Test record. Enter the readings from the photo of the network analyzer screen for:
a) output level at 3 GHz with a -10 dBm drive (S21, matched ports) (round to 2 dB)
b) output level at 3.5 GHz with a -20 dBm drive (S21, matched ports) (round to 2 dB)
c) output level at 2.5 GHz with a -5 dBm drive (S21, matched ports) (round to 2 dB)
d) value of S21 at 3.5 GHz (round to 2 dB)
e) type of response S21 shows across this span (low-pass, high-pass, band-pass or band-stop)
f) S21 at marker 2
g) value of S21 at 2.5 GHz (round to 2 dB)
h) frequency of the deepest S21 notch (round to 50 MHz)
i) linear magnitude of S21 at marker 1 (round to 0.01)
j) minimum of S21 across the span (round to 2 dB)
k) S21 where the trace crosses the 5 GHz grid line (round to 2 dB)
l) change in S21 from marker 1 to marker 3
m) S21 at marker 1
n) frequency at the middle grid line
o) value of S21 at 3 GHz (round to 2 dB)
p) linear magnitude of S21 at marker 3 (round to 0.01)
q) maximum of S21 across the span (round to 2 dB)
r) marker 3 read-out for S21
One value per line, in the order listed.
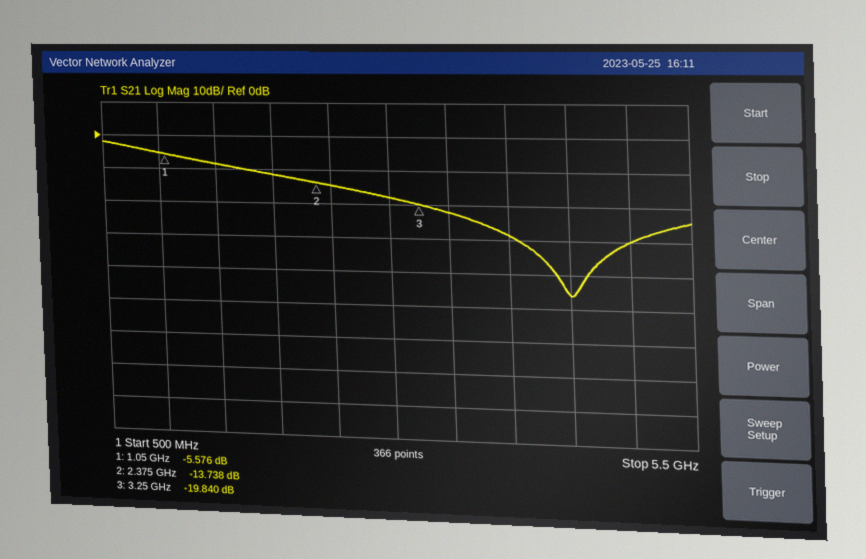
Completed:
-28 dBm
-42 dBm
-20 dBm
-22 dB
low-pass
-13.738 dB
-14 dB
4.50 GHz
0.53
-46 dB
-30 dB
-14.264 dB
-5.576 dB
3 GHz
-18 dB
0.10
-2 dB
-19.840 dB
